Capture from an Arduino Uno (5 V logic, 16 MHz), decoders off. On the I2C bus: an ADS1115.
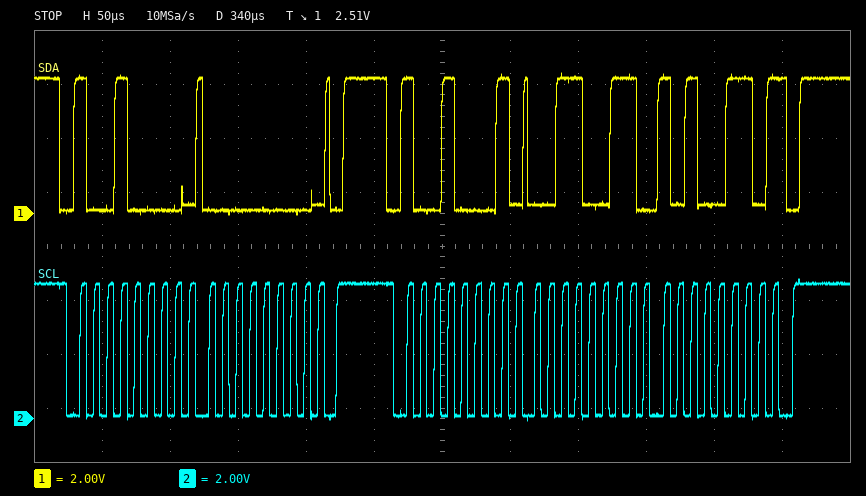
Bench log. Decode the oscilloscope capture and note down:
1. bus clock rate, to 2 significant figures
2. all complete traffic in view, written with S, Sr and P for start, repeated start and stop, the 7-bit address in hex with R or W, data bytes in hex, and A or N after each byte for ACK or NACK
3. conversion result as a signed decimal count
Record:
100 kHz
S 48W A 00 A P S 48R A 33 A A6 N P
13222
